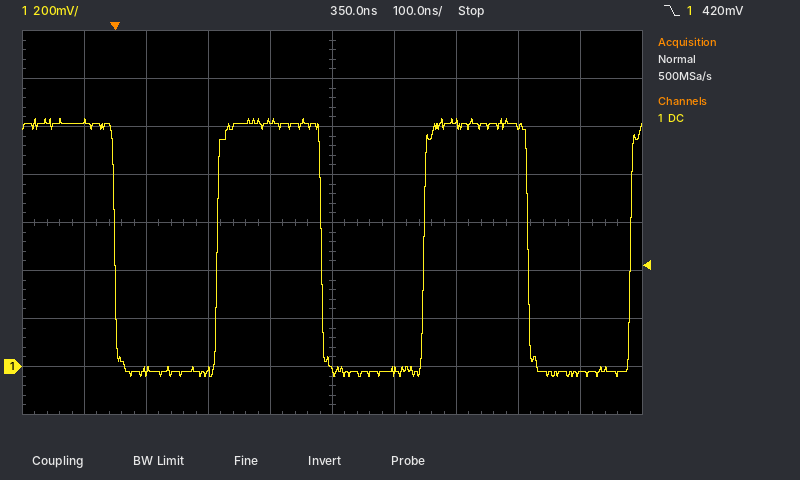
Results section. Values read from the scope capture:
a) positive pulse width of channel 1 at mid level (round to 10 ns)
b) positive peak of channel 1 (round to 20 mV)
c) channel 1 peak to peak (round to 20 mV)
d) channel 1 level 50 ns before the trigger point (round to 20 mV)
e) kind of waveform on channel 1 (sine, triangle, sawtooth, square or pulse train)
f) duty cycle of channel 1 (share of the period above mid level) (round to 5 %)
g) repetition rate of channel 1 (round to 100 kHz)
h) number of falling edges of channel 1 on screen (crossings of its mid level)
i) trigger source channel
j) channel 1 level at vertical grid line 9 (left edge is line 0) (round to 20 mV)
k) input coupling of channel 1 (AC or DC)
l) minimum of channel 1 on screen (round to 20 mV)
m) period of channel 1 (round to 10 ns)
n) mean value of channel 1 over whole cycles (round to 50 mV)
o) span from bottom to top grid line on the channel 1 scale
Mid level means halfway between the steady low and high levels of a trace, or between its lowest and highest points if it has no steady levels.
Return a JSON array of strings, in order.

["170 ns", "1.04 V", "1.08 V", "1.02 V", "square", "50 %", "3.0 MHz", "3", "channel 1", "-40 mV", "DC", "-40 mV", "330 ns", "500 mV", "1.6 V"]
